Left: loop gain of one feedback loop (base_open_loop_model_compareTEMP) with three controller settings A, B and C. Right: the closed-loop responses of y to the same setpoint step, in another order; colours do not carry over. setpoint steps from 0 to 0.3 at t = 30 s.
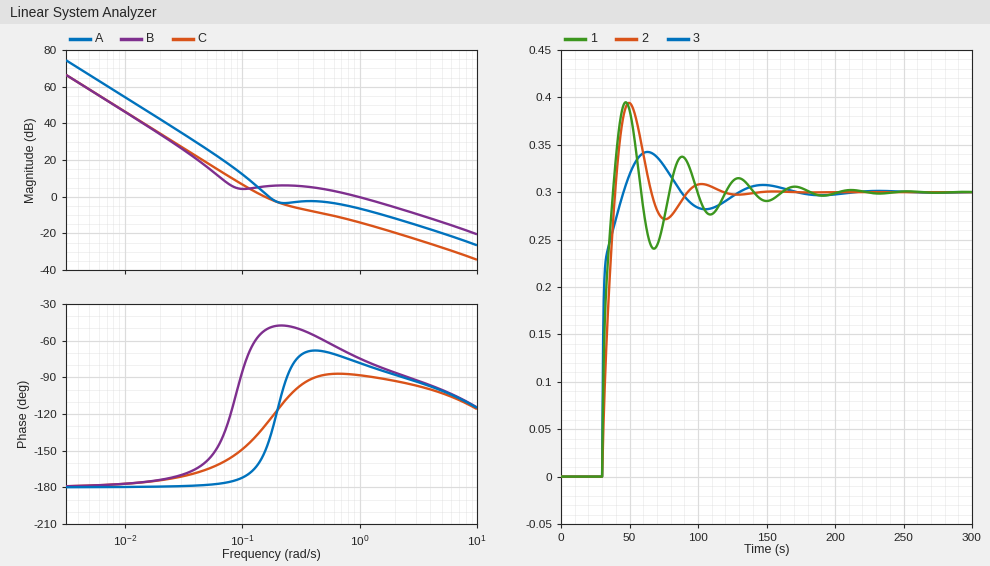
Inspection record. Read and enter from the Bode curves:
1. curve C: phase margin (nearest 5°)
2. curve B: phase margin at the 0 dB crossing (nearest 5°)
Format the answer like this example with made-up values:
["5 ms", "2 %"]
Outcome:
["50°", "105°"]
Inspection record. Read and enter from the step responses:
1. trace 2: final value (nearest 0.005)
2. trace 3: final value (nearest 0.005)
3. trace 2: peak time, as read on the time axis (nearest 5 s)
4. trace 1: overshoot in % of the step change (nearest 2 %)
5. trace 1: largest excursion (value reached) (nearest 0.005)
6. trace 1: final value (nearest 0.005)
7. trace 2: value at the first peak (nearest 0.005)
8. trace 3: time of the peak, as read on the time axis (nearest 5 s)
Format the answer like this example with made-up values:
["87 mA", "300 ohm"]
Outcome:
["0.300", "0.300", "50 s", "32 %", "0.395", "0.300", "0.395", "65 s"]
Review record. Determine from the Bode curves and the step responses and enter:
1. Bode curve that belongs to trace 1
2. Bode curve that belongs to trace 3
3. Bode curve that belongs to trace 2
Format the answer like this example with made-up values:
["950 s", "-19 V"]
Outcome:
["A", "B", "C"]
